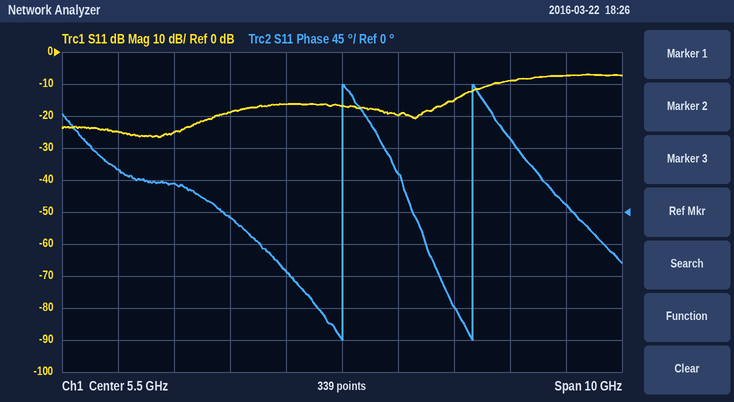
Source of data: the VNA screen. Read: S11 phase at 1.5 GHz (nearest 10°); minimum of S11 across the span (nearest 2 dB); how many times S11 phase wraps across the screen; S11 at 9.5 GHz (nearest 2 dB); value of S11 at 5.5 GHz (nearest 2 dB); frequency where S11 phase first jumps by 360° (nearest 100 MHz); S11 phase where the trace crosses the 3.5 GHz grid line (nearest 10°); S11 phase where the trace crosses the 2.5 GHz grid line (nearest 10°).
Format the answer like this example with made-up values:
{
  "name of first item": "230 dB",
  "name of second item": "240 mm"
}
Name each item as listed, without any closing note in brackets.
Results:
{
  "S11 phase at 1.5 GHz": "60°",
  "minimum of S11 across the span": "-26 dB",
  "how many times S11 phase wraps across the screen": "2",
  "S11 at 9.5 GHz": "-8 dB",
  "value of S11 at 5.5 GHz": "-16 dB",
  "frequency where S11 phase first jumps by 360°": "5.5 GHz",
  "S11 phase where the trace crosses the 3.5 GHz grid line": "-10°",
  "S11 phase where the trace crosses the 2.5 GHz grid line": "40°"
}
